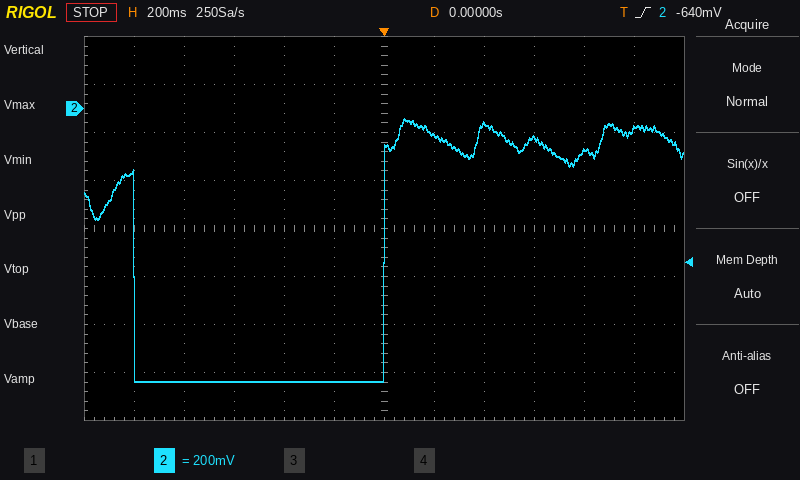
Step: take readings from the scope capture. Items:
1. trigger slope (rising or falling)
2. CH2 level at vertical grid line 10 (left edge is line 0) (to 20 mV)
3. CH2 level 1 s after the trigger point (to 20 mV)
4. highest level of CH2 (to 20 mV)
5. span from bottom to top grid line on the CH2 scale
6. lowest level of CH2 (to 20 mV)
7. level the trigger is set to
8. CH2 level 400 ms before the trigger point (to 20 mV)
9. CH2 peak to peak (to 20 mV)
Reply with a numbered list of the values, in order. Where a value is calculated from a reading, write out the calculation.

1. rising
2. -180 mV
3. -80 mV
4. -40 mV
5. 1.6 V
6. -1.14 V
7. -640 mV
8. -1.14 V
9. -40 mV − (-1.14 V) = 1.10 V
